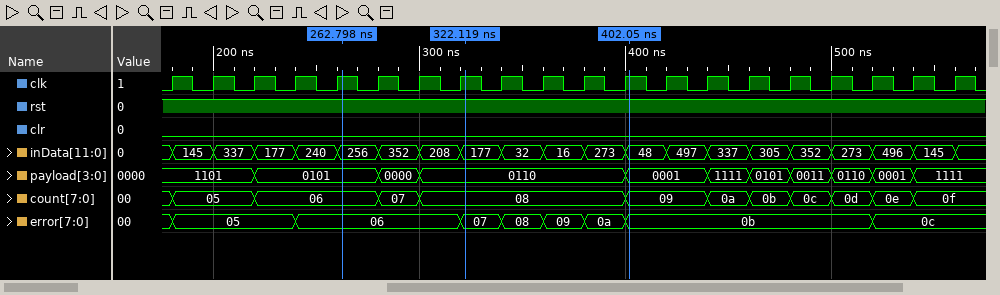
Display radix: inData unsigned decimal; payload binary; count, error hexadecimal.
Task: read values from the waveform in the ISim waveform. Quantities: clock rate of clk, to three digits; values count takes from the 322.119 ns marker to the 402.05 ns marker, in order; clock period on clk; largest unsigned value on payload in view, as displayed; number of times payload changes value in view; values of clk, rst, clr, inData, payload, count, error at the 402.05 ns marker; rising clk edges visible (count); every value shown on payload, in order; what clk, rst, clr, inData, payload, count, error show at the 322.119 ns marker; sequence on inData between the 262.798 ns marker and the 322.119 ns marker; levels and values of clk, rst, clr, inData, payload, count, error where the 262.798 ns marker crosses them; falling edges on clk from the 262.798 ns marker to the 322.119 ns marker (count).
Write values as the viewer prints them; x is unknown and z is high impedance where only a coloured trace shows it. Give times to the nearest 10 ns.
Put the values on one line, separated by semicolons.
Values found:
50.0 MHz; 08, 09; 20 ns; 1111; 10; clk=1, rst=1, clr=0, inData=48, payload=0001, count=09, error=0b; 20; 1101, 0101, 0000, 0110, 0001, 1111, 0101, 0011, 0110, 0001, 1111; clk=1, rst=1, clr=0, inData=177, payload=0110, count=08, error=07; 256, 352, 208, 177; clk=1, rst=1, clr=0, inData=256, payload=0101, count=06, error=06; 3
